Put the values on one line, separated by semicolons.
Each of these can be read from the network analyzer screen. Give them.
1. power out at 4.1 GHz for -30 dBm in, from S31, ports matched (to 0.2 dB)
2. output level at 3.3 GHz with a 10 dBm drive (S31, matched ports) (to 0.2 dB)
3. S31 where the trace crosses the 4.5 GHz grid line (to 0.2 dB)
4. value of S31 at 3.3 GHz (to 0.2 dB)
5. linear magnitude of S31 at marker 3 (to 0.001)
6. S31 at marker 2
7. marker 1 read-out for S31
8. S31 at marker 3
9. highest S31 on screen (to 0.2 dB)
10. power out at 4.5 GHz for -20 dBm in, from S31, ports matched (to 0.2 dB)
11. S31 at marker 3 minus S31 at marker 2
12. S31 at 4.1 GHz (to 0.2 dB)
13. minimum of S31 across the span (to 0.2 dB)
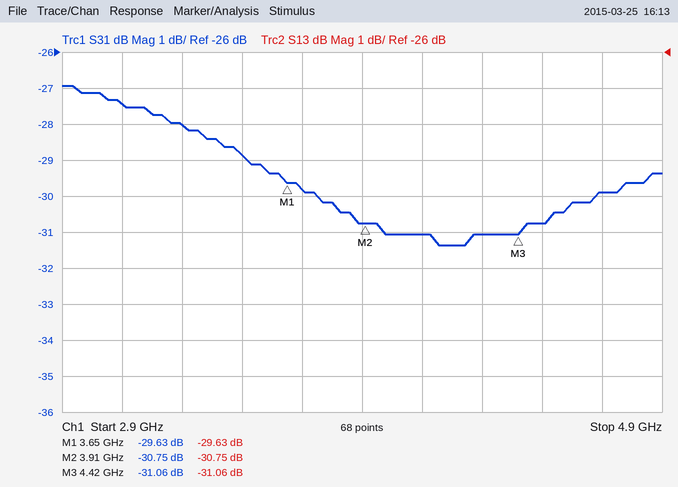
-61.0 dBm; -18.0 dBm; -30.8 dB; -28.0 dB; 0.028; -30.75 dB; -29.63 dB; -31.06 dB; -27.0 dB; -50.8 dBm; -0.31 dB; -31.0 dB; -31.4 dB
